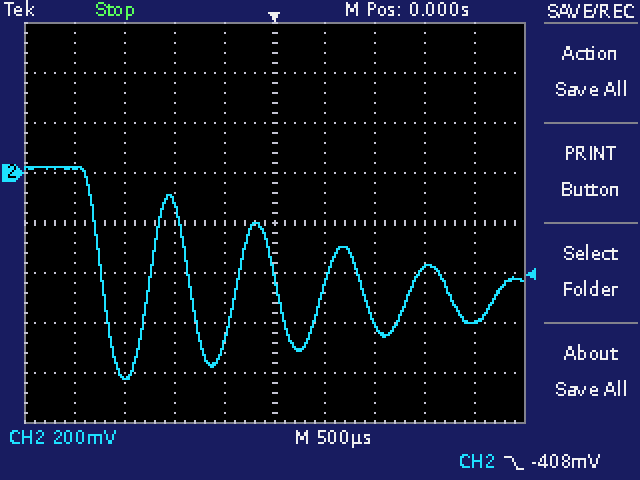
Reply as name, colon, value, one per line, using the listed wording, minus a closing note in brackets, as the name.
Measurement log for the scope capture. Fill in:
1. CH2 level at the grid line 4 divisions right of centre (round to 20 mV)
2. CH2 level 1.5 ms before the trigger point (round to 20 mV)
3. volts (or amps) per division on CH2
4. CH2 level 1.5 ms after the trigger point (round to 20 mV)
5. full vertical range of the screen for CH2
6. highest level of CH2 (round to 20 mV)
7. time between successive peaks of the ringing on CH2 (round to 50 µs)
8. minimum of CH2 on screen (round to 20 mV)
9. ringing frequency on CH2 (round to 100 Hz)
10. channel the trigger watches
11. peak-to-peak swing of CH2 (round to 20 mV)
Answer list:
CH2 level at the grid line 4 divisions right of centre: -600 mV
CH2 level 1.5 ms before the trigger point: -820 mV
volts (or amps) per division on CH2: 200 mV
CH2 level 1.5 ms after the trigger point: -380 mV
full vertical range of the screen for CH2: 1.6 V
highest level of CH2: 20 mV
time between successive peaks of the ringing on CH2: 850 µs
minimum of CH2 on screen: -820 mV
ringing frequency on CH2: 1.2 kHz
channel the trigger watches: CH2
peak-to-peak swing of CH2: 840 mV
